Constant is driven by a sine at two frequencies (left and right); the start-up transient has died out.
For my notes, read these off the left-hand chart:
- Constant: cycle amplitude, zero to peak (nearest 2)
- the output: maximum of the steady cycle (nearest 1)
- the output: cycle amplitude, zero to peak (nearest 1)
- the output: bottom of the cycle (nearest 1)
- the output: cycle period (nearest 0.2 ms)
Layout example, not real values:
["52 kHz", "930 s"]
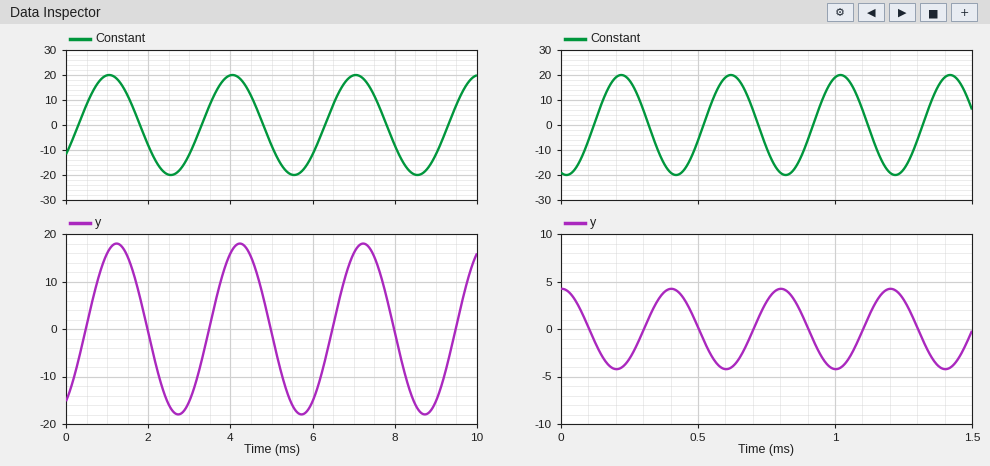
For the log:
["20", "18", "18", "-18", "3.0 ms"]
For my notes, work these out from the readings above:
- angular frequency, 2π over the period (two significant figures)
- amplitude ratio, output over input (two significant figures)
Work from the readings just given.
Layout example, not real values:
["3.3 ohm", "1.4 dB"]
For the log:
["2.1 rad/ms", "0.90"]
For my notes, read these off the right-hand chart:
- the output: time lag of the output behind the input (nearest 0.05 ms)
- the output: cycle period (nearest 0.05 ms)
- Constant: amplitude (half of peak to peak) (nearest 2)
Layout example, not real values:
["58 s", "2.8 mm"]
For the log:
["0.20 ms", "0.40 ms", "20"]
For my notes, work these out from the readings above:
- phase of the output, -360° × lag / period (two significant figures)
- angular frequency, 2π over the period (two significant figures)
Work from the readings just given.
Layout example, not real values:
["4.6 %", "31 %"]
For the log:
["-180°", "16 rad/ms"]
